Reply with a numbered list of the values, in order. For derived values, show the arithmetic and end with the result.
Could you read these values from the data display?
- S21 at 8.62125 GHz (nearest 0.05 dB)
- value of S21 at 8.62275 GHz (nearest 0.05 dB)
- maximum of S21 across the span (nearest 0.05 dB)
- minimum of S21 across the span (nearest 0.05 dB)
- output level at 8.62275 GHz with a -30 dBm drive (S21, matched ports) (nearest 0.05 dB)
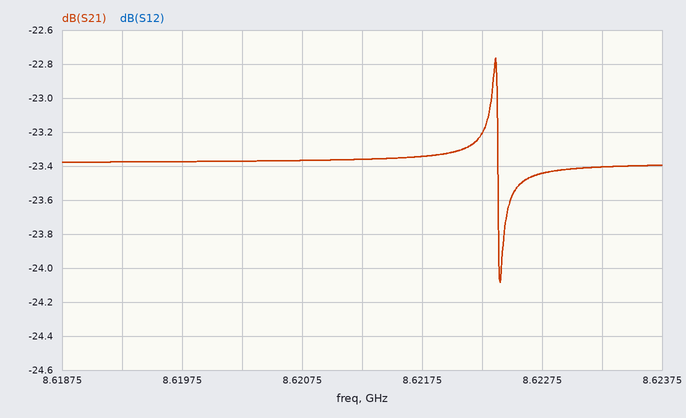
1. -23.35 dB
2. -23.45 dB
3. -22.75 dB
4. -24.10 dB
5. -30 dBm + (-23.45 dB) = -53.45 dBm
